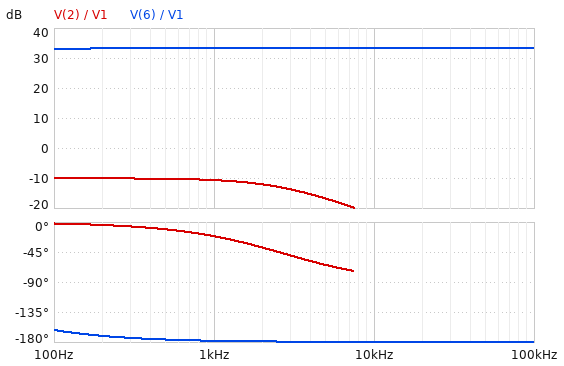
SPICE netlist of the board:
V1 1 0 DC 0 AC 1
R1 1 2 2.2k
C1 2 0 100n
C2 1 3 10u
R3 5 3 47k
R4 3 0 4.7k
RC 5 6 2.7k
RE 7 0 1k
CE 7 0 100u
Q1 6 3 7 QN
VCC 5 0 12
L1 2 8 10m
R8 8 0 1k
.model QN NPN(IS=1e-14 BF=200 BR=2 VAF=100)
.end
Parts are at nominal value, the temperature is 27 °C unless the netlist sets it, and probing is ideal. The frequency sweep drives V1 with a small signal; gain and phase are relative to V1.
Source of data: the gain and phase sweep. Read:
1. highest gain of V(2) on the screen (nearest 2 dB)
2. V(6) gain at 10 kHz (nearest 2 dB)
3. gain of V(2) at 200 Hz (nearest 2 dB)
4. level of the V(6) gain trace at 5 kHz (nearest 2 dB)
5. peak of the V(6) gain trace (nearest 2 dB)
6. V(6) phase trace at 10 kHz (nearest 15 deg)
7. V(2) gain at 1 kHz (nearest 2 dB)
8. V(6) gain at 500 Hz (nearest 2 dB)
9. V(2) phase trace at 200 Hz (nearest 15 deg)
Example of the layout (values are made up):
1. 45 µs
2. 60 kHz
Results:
1. -10 dB
2. 34 dB
3. -10 dB
4. 34 dB
5. 34 dB
6. -180 deg
7. -10 dB
8. 34 dB
9. 0 deg
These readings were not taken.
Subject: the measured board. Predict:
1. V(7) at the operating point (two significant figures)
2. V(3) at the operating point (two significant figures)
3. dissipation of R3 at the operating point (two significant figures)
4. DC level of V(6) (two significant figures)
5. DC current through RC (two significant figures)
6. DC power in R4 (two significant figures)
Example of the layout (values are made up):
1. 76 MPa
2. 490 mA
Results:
1. 450 mV
2. 1.1 V
3. 2.5 mW
4. 11 V
5. 450 µA
6. 250 µW
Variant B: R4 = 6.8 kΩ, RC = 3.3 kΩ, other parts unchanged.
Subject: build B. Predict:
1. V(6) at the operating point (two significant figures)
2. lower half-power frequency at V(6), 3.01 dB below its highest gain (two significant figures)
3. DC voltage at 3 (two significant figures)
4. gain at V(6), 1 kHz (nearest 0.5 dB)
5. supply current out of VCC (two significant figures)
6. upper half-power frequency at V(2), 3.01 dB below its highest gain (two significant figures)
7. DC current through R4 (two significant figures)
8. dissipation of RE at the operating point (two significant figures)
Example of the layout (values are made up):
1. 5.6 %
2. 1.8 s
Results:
1. 9.2 V
2. 55 Hz
3. 1.5 V
4. 40.5 dB
5. 1.1 mA
6. 2.6 kHz
7. 220 µA
8. 710 µW
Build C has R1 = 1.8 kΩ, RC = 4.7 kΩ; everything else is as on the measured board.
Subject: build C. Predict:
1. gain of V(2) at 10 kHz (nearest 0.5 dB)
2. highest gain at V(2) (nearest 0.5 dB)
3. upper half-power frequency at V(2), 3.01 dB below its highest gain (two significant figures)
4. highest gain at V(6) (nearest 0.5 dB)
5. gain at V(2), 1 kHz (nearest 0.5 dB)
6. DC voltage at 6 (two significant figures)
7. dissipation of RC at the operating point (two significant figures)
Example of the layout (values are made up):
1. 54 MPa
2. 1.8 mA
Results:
1. -20.5 dB
2. -9.0 dB
3. 2.8 kHz
4. 38.0 dB
5. -9.5 dB
6. 9.9 V
7. 940 µW
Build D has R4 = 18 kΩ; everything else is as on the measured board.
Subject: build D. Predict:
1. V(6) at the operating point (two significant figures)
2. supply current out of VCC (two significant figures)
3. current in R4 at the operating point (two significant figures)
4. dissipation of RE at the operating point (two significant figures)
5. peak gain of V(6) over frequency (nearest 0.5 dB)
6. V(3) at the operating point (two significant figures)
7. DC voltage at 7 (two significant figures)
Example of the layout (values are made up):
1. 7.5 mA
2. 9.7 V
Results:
1. 5.3 V
2. 2.7 mA
3. 180 µA
4. 6.2 mW
5. 47.5 dB
6. 3.2 V
7. 2.5 V
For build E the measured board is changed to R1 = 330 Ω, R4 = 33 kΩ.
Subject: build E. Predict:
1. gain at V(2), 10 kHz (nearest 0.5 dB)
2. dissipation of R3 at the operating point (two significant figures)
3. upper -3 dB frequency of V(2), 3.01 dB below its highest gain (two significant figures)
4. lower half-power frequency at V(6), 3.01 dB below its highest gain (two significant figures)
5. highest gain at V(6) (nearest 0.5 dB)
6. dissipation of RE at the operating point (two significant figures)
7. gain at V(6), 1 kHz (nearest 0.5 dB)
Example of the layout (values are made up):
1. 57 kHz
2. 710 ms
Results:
1. -7.0 dB
2. 1.4 mW
3. 7.3 kHz
4. 710 Hz
5. 29.0 dB
6. 11 mW
7. 27.0 dB
